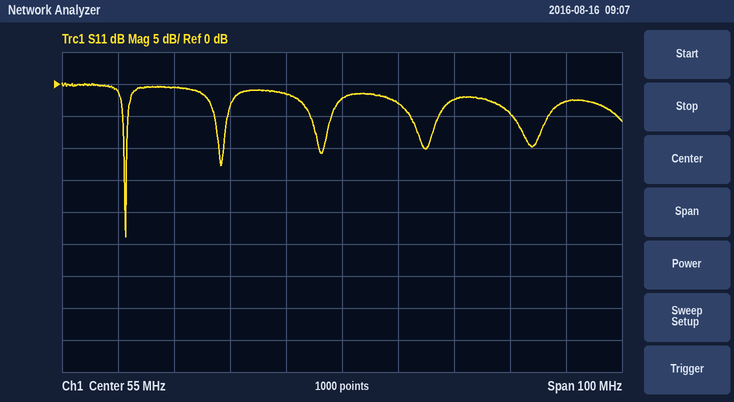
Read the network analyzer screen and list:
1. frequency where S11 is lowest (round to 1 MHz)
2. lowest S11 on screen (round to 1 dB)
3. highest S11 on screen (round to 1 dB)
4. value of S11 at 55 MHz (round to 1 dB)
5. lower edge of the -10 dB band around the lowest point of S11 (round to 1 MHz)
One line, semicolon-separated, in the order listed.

16 MHz; -24 dB; 0 dB; -2 dB; 16 MHz
